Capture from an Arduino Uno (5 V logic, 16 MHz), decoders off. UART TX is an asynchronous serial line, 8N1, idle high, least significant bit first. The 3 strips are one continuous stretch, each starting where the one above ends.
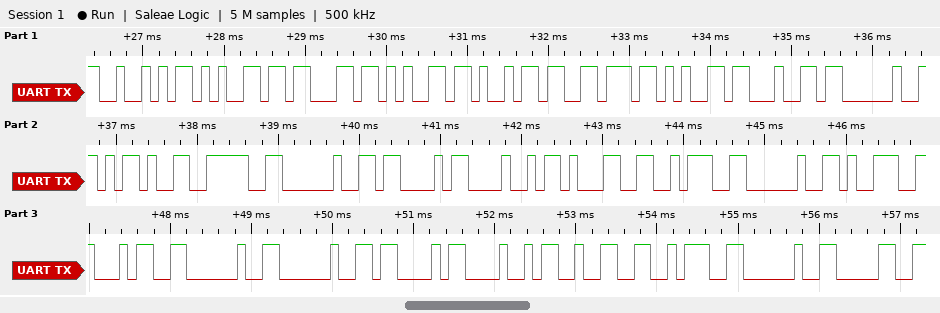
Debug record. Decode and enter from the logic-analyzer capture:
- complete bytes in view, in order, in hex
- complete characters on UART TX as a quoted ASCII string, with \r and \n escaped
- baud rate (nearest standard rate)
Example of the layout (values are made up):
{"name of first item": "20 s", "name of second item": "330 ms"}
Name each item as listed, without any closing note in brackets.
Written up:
{"complete bytes in view, in order, in hex": "52 65 63 65 69 76 65 64 20 2D 3E 20 43 48 31 3A 20 39 34 20 20 43 48 32 3A 20 30", "complete characters on UART TX as a quoted ASCII string, with \\r and \\n escaped": "\"Received -> CH1: 94  CH2: 0\"", "baud rate": "9600 baud"}
